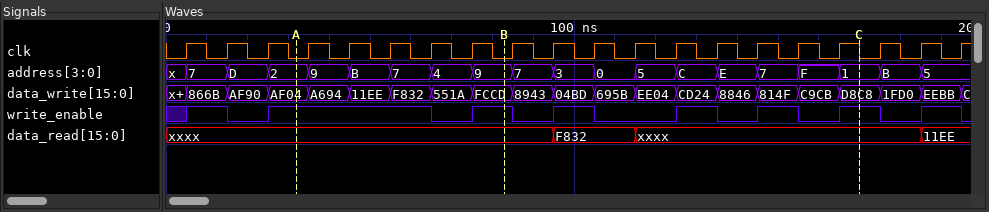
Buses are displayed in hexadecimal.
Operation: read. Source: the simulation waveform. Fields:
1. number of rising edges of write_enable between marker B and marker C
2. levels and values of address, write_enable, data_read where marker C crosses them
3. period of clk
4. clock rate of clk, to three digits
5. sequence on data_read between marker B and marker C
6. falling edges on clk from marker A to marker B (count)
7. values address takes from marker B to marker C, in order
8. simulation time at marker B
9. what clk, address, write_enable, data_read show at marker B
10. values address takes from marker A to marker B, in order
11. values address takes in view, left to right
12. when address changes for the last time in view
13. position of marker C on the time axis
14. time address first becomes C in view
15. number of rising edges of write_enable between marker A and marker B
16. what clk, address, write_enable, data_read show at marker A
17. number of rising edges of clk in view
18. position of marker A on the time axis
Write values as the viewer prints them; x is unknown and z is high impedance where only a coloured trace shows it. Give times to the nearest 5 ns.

4
address=1, write_enable=1, data_read=xxxx
10 ns
100 MHz
xxxx, F832, xxxx
5
9, 7, 3, 0, 5, C, E, 7, F, 1
85 ns
clk=0, address=9, write_enable=1, data_read=xxxx
2, 9, B, 7, 4, 9
x, 7, D, 2, 9, B, 7, 4, 9, 7, 3, 0, 5, C, E, 7, F, 1, B, 5
185 ns
170 ns
125 ns
1
clk=0, address=2, write_enable=1, data_read=xxxx
20
30 ns
